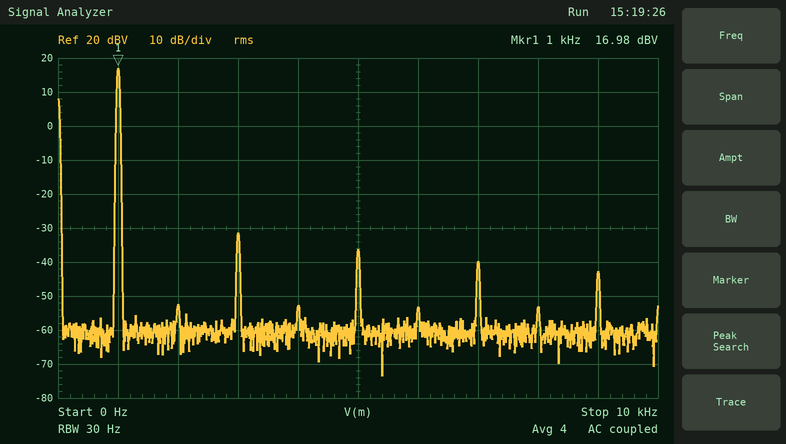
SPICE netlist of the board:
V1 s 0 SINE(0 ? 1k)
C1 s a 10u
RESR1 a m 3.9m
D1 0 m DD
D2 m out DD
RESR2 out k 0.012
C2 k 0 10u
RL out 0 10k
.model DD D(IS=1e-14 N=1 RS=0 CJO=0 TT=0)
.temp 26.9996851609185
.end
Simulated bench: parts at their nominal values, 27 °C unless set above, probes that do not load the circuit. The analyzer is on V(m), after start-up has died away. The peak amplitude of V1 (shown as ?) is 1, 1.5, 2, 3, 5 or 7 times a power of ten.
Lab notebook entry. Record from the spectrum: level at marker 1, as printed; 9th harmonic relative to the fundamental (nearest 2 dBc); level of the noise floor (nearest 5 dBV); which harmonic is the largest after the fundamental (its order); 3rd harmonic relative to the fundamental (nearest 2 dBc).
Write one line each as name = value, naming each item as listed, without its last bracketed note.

level at marker 1, as printed = 16.98 dBV
9th harmonic relative to the fundamental = -60 dBc
level of the noise floor = -60 dBV
which harmonic is the largest after the fundamental = 3
3rd harmonic relative to the fundamental = -48 dBc
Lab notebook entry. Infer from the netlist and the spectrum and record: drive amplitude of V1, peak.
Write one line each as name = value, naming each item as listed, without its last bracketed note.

drive amplitude of V1, peak = 10 V
